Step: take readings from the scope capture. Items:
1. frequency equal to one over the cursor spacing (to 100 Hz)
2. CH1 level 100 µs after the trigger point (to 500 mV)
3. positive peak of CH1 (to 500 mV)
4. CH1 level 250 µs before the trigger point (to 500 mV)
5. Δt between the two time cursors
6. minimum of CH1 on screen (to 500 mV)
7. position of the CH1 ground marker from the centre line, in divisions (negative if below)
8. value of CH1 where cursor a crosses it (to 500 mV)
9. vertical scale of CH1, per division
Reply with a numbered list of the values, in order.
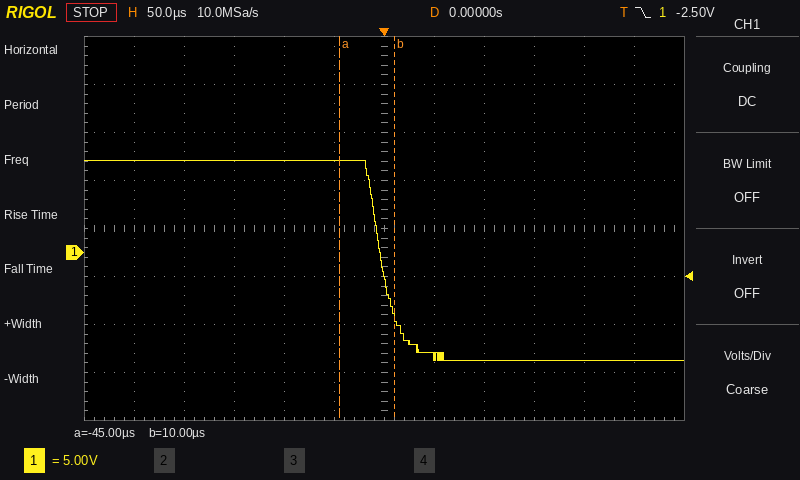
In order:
1. 18.2 kHz
2. -11.0 V
3. 9.5 V
4. 9.5 V
5. 55 µs
6. -11.0 V
7. -0.5 div
8. 9.5 V
9. 5 V
